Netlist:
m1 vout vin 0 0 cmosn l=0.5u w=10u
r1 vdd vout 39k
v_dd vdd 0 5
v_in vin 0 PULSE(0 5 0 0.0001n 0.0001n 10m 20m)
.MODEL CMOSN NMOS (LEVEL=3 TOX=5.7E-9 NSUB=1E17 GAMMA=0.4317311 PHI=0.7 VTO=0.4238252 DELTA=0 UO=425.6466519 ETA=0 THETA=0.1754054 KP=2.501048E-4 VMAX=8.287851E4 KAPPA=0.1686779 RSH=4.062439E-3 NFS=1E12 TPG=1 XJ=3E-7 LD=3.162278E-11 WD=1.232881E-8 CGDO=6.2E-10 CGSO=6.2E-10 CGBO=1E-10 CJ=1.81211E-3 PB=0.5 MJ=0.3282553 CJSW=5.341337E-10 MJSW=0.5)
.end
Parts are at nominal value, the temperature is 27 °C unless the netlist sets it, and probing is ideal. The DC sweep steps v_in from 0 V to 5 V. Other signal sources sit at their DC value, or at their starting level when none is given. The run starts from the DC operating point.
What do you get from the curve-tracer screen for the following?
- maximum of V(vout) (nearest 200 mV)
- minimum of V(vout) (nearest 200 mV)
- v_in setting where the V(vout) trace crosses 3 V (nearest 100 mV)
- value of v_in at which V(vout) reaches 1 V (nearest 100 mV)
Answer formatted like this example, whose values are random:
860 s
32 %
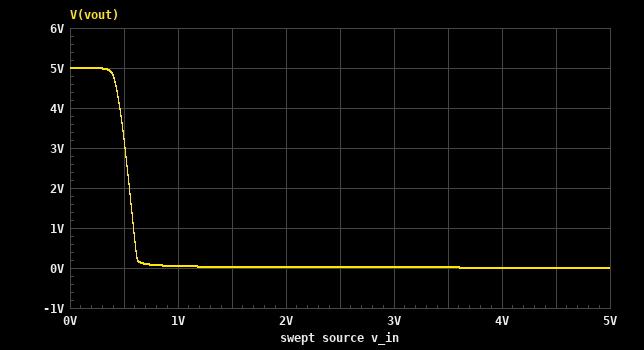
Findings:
5.0 V
0 V
500 mV
600 mV
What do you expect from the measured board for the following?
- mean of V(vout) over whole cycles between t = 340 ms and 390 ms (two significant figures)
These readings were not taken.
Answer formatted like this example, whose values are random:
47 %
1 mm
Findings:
2.5 V
